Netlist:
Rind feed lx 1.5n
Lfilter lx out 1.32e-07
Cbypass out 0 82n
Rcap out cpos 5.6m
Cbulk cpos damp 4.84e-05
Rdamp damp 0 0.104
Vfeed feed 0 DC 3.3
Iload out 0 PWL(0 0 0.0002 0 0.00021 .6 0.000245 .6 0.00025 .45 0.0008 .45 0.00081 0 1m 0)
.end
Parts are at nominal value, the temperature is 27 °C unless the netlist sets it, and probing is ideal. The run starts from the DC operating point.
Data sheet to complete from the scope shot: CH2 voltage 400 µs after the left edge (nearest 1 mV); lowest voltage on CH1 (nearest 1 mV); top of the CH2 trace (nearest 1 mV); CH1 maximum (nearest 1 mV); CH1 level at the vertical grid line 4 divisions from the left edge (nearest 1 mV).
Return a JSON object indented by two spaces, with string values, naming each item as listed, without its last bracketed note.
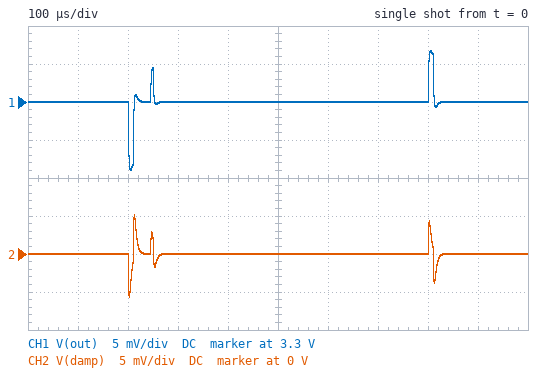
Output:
{
  "CH2 voltage 400 µs after the left edge": "0 V",
  "lowest voltage on CH1": "3.291 V",
  "top of the CH2 trace": "5 mV",
  "CH1 maximum": "3.307 V",
  "CH1 level at the vertical grid line 4 divisions from the left edge": "3.300 V"
}
